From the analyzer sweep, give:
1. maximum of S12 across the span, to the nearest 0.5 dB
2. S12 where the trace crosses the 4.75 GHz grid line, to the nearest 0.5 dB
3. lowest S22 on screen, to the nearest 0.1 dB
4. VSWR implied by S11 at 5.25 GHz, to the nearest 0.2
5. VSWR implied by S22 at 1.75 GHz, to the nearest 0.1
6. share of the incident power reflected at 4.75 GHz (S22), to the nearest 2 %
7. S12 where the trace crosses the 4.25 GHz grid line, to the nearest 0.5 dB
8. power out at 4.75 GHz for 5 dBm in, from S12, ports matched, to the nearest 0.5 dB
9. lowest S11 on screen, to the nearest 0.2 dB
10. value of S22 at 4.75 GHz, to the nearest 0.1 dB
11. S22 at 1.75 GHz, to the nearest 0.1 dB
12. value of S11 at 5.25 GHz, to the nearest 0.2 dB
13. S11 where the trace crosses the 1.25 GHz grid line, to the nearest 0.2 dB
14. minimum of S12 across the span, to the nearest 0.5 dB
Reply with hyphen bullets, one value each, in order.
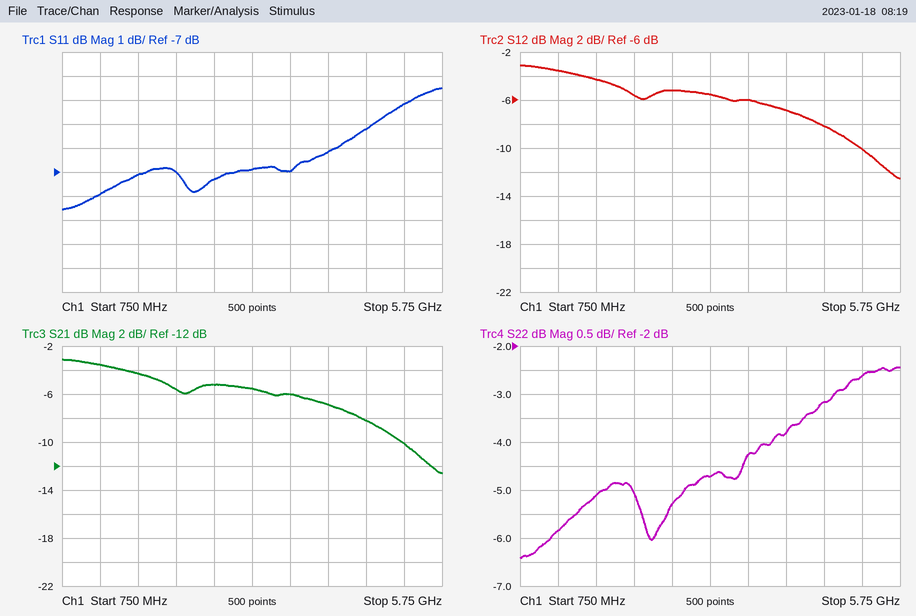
- -3.0 dB
- -8.0 dB
- -6.4 dB
- 4.2
- 3.5
- 48 %
- -7.0 dB
- -3.0 dBm
- -8.6 dB
- -3.2 dB
- -5.1 dB
- -4.2 dB
- -8.0 dB
- -12.5 dB
